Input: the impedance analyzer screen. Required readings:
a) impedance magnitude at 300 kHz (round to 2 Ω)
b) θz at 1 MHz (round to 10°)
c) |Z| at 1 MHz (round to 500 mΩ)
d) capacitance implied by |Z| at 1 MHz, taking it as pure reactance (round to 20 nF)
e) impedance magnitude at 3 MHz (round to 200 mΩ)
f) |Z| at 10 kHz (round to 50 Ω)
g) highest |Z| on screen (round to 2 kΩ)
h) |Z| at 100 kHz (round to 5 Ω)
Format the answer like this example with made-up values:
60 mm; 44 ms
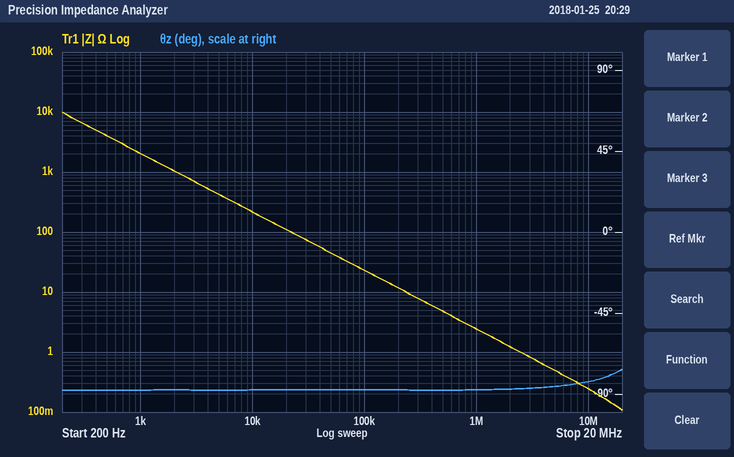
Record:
8 Ω; -90°; 2.5 Ω; 60 nF; 800 mΩ; 200 Ω; 10 kΩ; 25 Ω
